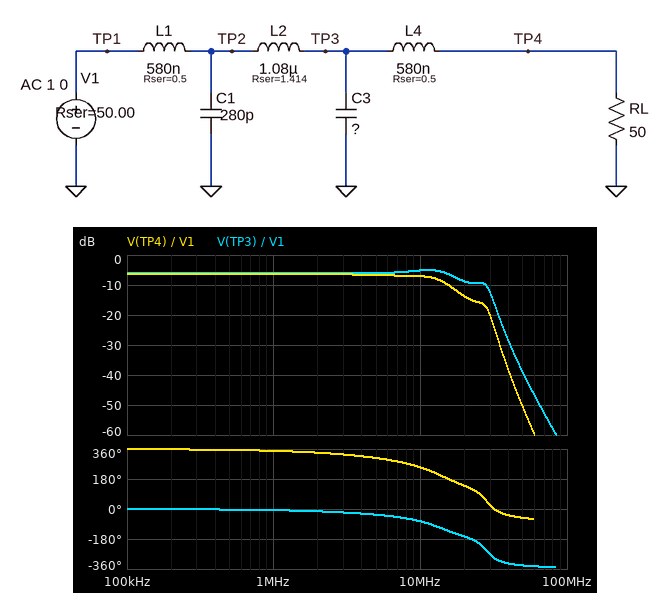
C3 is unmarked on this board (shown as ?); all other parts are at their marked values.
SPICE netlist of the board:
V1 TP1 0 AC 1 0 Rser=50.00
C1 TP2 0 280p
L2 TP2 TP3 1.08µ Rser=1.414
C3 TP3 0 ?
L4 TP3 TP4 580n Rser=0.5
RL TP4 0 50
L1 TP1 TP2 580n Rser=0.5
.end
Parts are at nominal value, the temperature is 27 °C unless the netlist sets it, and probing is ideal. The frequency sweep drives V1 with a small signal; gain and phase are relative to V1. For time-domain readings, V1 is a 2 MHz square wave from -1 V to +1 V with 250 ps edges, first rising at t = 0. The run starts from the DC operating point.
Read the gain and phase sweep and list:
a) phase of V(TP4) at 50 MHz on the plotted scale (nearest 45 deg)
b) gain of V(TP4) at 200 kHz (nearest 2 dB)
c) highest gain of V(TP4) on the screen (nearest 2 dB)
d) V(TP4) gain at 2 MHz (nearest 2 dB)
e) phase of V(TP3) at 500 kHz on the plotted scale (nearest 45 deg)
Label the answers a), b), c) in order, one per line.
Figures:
a) -45 deg
b) -6 dB
c) -6 dB
d) -6 dB
e) 0 deg
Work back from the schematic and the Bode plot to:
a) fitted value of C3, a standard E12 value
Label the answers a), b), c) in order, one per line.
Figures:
a) 82 pF
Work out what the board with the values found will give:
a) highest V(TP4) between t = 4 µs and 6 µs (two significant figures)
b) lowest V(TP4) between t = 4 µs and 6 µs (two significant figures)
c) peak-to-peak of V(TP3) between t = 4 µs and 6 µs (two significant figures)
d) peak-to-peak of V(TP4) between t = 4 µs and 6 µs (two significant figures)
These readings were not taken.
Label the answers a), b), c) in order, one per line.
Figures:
a) 510 mV
b) -510 mV
c) 1.3 V
d) 1.0 V
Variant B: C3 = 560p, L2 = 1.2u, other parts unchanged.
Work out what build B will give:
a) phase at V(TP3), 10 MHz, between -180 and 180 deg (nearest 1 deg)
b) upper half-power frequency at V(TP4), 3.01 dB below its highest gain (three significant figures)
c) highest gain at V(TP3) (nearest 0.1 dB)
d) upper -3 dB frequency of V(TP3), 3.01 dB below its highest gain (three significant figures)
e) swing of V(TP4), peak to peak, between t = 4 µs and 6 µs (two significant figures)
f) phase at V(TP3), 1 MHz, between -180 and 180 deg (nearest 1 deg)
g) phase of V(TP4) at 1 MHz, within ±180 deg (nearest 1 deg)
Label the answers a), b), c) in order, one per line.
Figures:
a) -139 deg
b) 12.1 MHz
c) -5.7 dB
d) 14.1 MHz
e) 1.2 V
f) -12 deg
g) -16 deg
